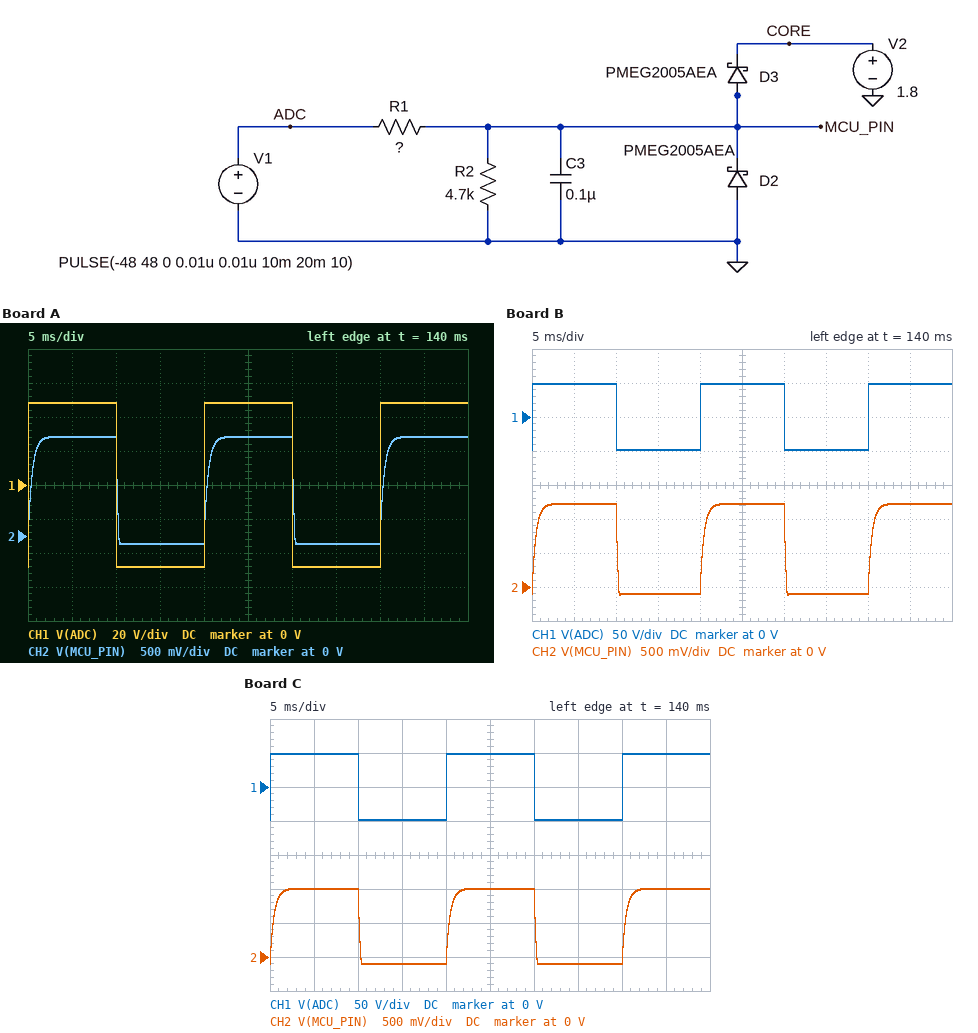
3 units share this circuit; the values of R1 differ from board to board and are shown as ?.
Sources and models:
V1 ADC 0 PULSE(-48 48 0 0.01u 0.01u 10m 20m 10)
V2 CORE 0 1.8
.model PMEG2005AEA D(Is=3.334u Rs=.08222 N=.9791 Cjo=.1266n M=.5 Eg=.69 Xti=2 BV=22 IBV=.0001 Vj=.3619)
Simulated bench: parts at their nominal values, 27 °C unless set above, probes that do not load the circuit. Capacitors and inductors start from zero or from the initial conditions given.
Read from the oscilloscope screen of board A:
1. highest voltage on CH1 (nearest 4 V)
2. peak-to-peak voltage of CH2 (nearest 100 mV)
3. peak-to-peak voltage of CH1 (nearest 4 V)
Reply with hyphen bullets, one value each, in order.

- 48 V
- 1.6 V
- 96 V
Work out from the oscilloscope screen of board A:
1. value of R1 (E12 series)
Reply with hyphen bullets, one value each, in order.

- 150 kΩ
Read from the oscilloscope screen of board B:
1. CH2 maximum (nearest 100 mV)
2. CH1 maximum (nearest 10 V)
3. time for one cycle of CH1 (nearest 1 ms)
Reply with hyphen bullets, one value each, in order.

- 1.2 V
- 50 V
- 20 ms
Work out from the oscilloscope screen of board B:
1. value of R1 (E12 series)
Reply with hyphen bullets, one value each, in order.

- 180 kΩ
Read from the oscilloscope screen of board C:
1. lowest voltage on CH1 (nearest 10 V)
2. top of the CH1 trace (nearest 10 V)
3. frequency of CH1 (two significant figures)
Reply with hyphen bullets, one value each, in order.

- -50 V
- 50 V
- 50 Hz
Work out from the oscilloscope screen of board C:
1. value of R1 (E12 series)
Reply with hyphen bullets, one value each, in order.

- 220 kΩ
